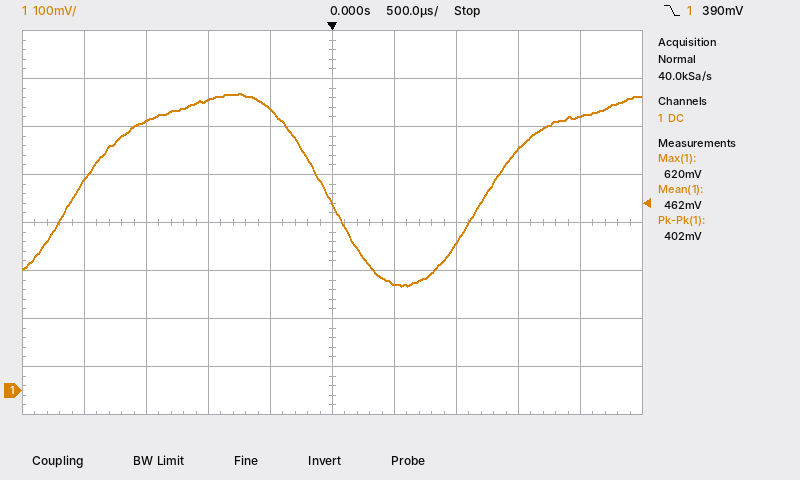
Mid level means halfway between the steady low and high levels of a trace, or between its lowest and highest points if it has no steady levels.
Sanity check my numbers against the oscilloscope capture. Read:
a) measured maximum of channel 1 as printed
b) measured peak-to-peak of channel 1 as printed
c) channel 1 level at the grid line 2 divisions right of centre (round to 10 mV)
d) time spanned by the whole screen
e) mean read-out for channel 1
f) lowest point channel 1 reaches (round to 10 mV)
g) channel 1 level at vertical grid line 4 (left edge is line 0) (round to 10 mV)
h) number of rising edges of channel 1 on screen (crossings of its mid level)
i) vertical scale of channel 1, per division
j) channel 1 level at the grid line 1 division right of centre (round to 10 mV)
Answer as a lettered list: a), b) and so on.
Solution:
a) 620 mV
b) 402 mV
c) 310 mV
d) 5 ms
e) 462 mV
f) 220 mV
g) 590 mV
h) 2
i) 100 mV
j) 220 mV
